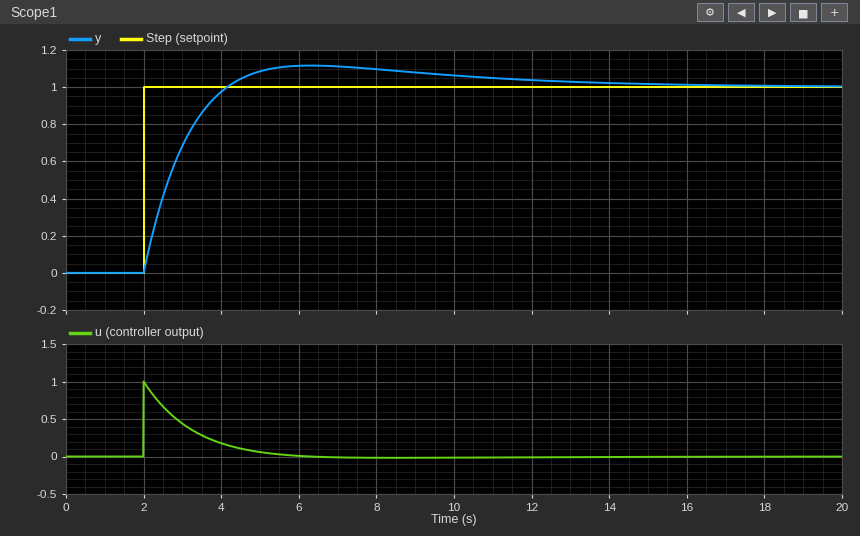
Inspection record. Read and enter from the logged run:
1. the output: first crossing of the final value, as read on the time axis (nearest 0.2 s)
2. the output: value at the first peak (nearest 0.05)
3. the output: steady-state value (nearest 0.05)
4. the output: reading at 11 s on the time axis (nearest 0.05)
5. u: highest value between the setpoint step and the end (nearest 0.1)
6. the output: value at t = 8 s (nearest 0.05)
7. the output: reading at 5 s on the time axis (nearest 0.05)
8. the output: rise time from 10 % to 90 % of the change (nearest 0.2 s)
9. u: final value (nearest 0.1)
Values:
4.2 s
1.10
1.00
1.05
1.0
1.10
1.10
1.6 s
0.0
